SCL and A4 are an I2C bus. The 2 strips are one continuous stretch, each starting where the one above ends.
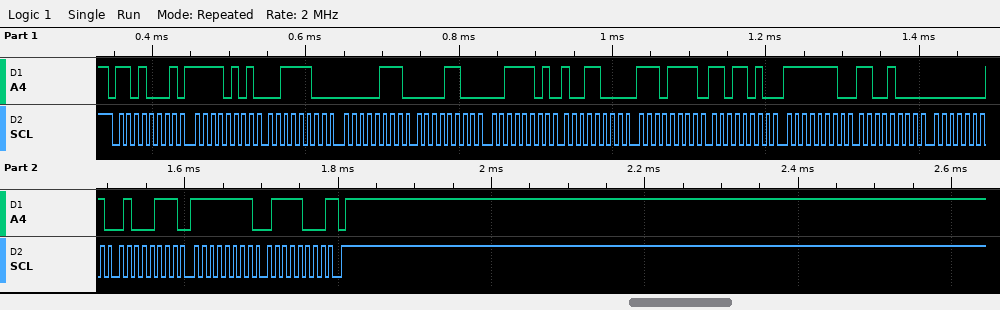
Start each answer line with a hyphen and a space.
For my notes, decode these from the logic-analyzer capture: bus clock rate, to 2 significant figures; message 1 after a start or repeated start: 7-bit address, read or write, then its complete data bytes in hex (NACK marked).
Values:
- 100 kHz
- 0x68 read: F5 3C 07 0C 3D 98 EF DA FE C8 01 47 FF 78 NACK
